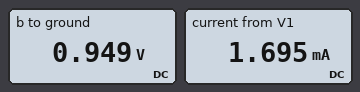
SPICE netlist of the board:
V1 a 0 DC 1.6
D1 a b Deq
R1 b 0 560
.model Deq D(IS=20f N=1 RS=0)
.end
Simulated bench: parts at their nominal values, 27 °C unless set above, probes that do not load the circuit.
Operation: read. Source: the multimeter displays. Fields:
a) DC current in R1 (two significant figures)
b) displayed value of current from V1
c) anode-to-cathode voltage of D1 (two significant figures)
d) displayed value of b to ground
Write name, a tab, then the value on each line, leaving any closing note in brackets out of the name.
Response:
DC current in R1	1.7 mA
displayed value of current from V1	1.695 mA
anode-to-cathode voltage of D1	650 mV
displayed value of b to ground	0.949 V
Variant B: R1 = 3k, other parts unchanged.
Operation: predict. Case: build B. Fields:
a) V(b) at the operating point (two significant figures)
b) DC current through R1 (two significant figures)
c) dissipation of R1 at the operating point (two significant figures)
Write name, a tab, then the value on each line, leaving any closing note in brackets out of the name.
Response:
V(b) at the operating point	990 mV
DC current through R1	330 µA
dissipation of R1 at the operating point	330 µW
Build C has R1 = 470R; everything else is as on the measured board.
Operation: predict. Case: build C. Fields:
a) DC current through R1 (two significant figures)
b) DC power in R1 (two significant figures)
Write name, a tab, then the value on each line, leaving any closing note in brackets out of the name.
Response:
DC current through R1	2.0 mA
DC power in R1	1.9 mW
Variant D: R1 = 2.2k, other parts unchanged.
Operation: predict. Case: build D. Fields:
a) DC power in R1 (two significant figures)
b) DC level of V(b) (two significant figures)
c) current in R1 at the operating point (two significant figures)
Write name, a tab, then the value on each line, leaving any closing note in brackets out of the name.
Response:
DC power in R1	440 µW
DC level of V(b)	980 mV
current in R1 at the operating point	450 µA
